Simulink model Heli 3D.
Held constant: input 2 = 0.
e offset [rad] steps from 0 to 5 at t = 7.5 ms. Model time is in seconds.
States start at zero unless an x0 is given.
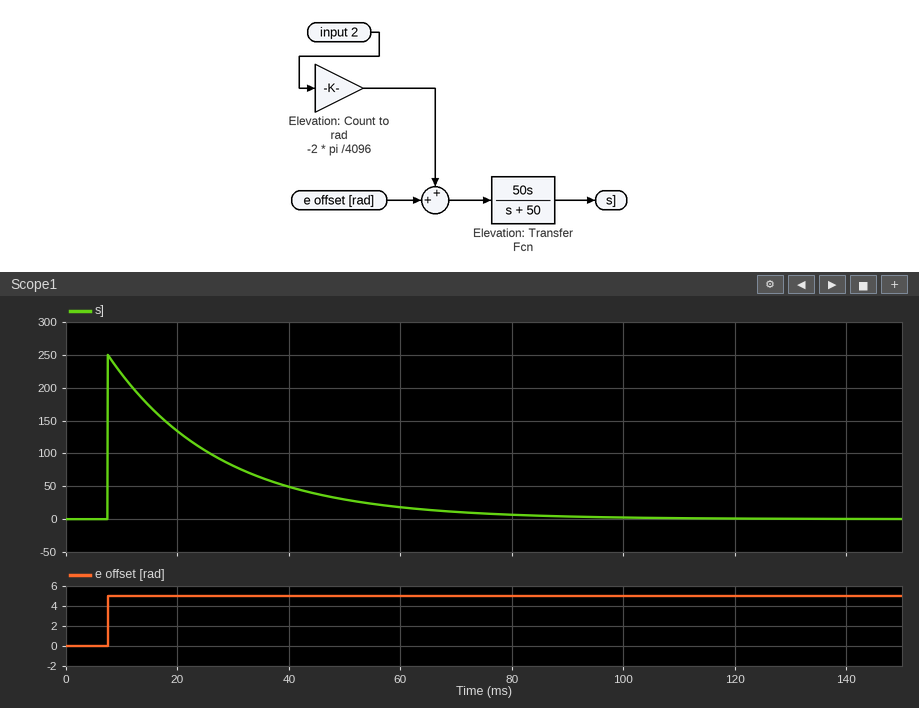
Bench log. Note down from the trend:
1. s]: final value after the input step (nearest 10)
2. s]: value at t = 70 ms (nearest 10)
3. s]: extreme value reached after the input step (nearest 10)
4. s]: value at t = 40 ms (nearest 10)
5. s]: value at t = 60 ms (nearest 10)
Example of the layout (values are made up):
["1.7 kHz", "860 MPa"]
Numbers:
["0", "10", "250", "50", "20"]
